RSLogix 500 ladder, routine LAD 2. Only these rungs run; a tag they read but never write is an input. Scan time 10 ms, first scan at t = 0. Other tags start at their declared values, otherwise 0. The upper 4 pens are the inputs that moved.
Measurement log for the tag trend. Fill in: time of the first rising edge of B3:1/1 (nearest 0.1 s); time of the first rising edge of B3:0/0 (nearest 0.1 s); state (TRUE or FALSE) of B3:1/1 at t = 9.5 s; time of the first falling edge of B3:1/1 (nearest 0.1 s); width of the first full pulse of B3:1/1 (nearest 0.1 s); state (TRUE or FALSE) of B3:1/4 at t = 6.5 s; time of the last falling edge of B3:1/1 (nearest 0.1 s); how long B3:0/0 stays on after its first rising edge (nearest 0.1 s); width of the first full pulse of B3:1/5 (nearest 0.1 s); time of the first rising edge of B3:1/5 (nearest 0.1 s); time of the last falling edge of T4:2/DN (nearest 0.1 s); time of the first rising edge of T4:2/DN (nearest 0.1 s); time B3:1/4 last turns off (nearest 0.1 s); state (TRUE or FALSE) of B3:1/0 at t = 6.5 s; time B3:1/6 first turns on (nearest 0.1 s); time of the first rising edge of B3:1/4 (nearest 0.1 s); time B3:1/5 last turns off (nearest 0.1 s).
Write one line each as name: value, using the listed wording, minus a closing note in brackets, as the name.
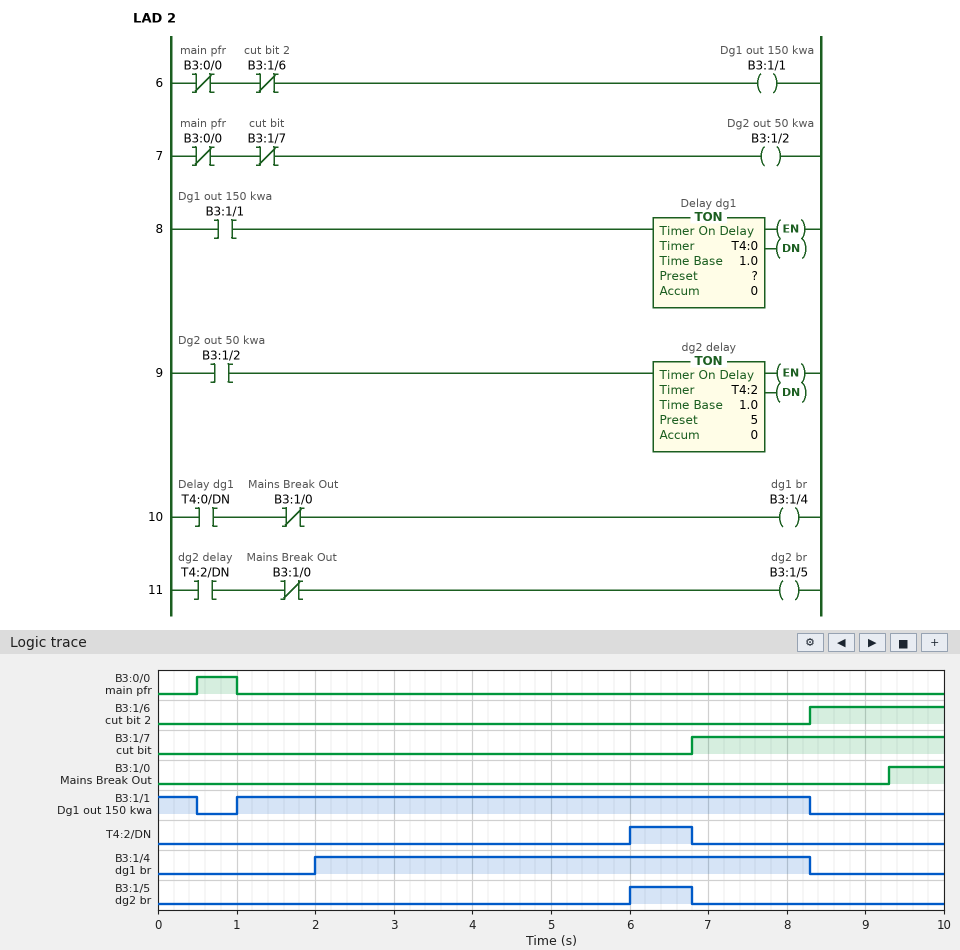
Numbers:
time of the first rising edge of B3:1/1: 1.0 s
time of the first rising edge of B3:0/0: 0.5 s
state (TRUE or FALSE) of B3:1/1 at t = 9.5 s: FALSE
time of the first falling edge of B3:1/1: 0.5 s
width of the first full pulse of B3:1/1: 7.3 s
state (TRUE or FALSE) of B3:1/4 at t = 6.5 s: TRUE
time of the last falling edge of B3:1/1: 8.3 s
how long B3:0/0 stays on after its first rising edge: 0.5 s
width of the first full pulse of B3:1/5: 0.8 s
time of the first rising edge of B3:1/5: 6.0 s
time of the last falling edge of T4:2/DN: 6.8 s
time of the first rising edge of T4:2/DN: 6.0 s
time B3:1/4 last turns off: 8.3 s
state (TRUE or FALSE) of B3:1/0 at t = 6.5 s: FALSE
time B3:1/6 first turns on: 8.3 s
time of the first rising edge of B3:1/4: 2.0 s
time B3:1/5 last turns off: 6.8 s
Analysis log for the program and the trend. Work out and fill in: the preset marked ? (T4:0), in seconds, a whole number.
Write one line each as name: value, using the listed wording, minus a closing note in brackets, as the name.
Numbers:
the preset marked ? (T4:0), in seconds, a whole number: 1 s
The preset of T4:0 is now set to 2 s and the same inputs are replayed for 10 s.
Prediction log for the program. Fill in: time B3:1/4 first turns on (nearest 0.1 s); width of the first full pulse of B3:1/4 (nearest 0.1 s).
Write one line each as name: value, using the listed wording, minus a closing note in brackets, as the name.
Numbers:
time B3:1/4 first turns on: 3.0 s
width of the first full pulse of B3:1/4: 5.3 s
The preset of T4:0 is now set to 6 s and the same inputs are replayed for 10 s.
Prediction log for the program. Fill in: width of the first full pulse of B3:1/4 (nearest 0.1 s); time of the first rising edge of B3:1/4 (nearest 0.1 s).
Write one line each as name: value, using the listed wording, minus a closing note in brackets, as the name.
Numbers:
width of the first full pulse of B3:1/4: 1.3 s
time of the first rising edge of B3:1/4: 7.0 s
